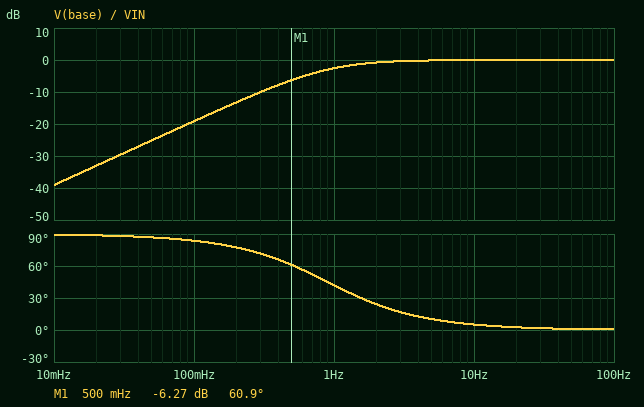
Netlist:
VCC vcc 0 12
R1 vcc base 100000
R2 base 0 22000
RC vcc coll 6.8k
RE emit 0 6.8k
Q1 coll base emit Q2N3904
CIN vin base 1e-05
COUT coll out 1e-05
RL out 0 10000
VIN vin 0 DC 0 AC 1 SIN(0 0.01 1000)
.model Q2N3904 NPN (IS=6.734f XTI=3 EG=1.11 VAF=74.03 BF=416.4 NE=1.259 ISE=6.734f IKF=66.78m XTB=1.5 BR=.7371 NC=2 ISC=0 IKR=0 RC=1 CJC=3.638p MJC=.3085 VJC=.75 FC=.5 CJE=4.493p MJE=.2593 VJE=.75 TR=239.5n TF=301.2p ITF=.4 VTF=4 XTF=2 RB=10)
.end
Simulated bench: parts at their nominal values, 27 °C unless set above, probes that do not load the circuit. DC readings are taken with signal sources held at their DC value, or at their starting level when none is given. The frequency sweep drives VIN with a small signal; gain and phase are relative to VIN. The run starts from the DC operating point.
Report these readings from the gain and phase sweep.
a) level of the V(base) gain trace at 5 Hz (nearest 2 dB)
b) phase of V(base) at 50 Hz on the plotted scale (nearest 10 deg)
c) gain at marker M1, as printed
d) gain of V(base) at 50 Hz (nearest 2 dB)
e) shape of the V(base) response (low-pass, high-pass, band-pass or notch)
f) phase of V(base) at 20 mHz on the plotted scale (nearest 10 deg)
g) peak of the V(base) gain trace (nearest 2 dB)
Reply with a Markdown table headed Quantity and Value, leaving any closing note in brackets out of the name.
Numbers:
| Quantity | Value |
|---|---|
| level of the V(base) gain trace at 5 Hz | 0 dB |
| phase of V(base) at 50 Hz on the plotted scale | 0 deg |
| gain at marker M1, as printed | -6.27 dB |
| gain of V(base) at 50 Hz | 0 dB |
| shape of the V(base) response | high-pass |
| phase of V(base) at 20 mHz on the plotted scale | 90 deg |
| peak of the V(base) gain trace | 0 dB |
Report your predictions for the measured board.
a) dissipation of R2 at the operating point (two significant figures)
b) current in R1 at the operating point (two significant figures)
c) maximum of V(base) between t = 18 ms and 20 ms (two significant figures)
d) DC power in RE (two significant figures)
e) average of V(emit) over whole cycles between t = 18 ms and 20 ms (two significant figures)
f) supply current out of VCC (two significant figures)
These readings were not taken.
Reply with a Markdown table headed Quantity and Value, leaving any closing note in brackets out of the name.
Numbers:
| Quantity | Value |
|---|---|
| dissipation of R2 at the operating point | 210 µW |
| current in R1 at the operating point | 99 µA |
| maximum of V(base) between t = 18 ms and 20 ms | 2.1 V |
| DC power in RE | 330 µW |
| average of V(emit) over whole cycles between t = 18 ms and 20 ms | 1.5 V |
| supply current out of VCC | 320 µA |
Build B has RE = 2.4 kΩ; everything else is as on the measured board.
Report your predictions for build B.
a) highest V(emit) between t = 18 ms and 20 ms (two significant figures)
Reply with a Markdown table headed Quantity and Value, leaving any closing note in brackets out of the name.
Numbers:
| Quantity | Value |
|---|---|
| highest V(emit) between t = 18 ms and 20 ms | 1.4 V |
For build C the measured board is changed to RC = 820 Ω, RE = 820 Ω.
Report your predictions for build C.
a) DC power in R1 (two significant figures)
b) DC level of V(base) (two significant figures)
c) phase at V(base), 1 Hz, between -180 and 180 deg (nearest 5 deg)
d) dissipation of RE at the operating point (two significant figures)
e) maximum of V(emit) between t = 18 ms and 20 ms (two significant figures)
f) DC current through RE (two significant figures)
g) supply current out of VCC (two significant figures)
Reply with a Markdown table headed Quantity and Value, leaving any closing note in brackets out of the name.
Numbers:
| Quantity | Value |
|---|---|
| DC power in R1 | 1.0 mW |
| DC level of V(base) | 2.0 V |
| phase at V(base), 1 Hz, between -180 and 180 deg | 45 deg |
| dissipation of RE at the operating point | 2.1 mW |
| maximum of V(emit) between t = 18 ms and 20 ms | 1.3 V |
| DC current through RE | 1.6 mA |
| supply current out of VCC | 1.7 mA |
